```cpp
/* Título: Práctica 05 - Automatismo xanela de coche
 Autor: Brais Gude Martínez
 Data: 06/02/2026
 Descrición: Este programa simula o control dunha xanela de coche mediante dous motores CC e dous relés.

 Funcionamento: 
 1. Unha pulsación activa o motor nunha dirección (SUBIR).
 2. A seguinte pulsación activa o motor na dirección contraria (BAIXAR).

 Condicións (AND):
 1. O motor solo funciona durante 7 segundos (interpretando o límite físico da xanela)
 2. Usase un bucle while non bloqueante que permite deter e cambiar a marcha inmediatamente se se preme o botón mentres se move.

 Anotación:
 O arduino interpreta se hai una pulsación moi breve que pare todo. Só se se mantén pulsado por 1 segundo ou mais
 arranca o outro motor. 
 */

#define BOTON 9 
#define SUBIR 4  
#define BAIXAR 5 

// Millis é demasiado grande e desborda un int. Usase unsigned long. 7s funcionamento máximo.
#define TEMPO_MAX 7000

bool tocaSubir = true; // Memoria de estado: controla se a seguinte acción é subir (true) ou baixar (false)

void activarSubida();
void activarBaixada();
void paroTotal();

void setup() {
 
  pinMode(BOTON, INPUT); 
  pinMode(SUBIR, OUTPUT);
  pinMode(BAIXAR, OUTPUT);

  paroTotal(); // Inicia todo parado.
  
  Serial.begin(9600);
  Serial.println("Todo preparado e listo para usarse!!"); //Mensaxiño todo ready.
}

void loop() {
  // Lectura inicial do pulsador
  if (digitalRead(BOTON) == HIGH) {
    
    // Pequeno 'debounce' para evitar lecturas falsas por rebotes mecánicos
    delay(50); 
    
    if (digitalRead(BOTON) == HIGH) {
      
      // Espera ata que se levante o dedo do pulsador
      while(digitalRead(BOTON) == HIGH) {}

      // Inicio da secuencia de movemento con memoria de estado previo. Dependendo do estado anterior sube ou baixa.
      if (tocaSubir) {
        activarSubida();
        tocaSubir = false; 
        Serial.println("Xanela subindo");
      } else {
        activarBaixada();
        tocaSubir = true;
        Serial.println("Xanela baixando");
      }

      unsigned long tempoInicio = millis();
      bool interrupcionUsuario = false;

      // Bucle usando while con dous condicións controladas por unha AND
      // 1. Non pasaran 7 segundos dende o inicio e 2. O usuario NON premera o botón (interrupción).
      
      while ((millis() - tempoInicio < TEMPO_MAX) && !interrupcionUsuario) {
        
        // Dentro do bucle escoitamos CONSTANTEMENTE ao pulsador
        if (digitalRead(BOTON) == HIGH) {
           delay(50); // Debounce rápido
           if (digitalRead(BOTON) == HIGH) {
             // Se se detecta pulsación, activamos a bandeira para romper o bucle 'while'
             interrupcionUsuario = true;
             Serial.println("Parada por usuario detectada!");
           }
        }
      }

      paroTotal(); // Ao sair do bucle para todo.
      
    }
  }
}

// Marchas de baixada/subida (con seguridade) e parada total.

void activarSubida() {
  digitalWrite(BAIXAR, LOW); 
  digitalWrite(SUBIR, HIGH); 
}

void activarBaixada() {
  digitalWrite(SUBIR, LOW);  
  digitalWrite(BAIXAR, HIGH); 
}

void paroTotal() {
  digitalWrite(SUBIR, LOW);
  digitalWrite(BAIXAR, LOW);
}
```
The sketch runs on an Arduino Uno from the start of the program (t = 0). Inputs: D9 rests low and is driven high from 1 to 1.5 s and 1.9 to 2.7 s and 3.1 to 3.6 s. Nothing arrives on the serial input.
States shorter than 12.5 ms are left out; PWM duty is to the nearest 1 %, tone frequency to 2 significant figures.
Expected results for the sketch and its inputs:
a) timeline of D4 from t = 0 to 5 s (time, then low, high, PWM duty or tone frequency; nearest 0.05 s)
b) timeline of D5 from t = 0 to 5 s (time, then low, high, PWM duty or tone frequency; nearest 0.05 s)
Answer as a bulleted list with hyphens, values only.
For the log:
- 0 s low; 1.5 s high; 1.95 s low; 3.6 s high
- 0 s low; 2.7 s high; 3.15 s low
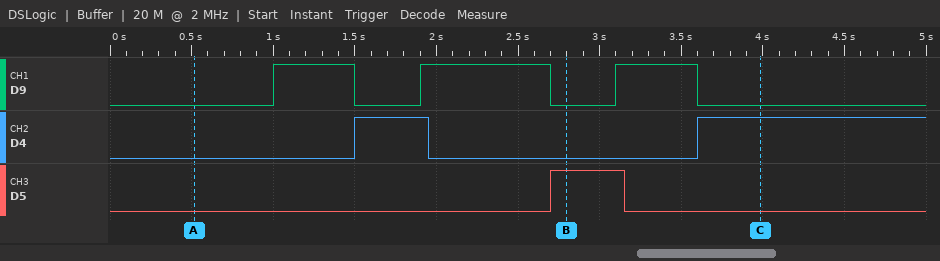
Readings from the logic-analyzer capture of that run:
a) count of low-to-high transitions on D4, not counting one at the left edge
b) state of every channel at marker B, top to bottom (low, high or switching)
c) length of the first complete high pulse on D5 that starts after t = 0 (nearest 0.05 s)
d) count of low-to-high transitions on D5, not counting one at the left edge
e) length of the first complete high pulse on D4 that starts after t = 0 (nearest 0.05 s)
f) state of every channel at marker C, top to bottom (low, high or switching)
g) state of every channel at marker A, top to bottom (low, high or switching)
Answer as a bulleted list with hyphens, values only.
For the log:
- 2
- D9 low, D4 low, D5 high
- 0.45 s
- 1
- 0.45 s
- D9 low, D4 high, D5 low
- D9 low, D4 low, D5 low
